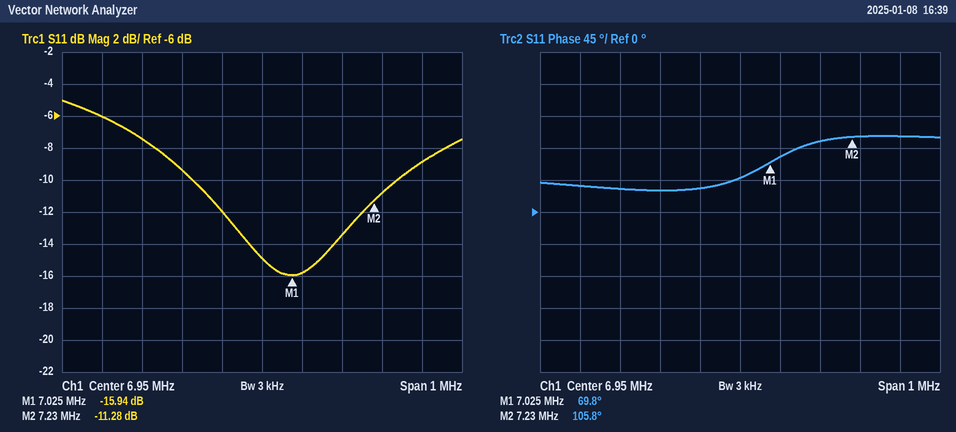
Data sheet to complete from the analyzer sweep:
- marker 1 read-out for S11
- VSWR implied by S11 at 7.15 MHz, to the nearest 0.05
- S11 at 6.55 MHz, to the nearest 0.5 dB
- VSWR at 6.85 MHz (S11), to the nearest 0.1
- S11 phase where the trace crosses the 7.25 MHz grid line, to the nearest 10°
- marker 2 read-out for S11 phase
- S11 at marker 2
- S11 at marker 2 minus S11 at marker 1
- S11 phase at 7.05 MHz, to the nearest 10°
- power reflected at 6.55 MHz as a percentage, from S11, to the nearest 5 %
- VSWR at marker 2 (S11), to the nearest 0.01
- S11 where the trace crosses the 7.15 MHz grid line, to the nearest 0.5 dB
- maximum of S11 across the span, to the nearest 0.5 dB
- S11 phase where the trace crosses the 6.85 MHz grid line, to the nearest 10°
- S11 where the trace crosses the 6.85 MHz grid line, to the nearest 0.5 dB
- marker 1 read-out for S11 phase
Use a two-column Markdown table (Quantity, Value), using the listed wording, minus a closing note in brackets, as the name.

| Quantity | Value |
|---|---|
| marker 1 read-out for S11 | -15.94 dB |
| VSWR implied by S11 at 7.15 MHz, to the nearest 0.05 | 1.55 |
| S11 at 6.55 MHz, to the nearest 0.5 dB | -6.0 dB |
| VSWR at 6.85 MHz (S11), to the nearest 0.1 | 1.7 |
| S11 phase where the trace crosses the 7.25 MHz grid line, to the nearest 10° | 110° |
| marker 2 read-out for S11 phase | 105.8° |
| S11 at marker 2 | -11.28 dB |
| S11 at marker 2 minus S11 at marker 1 | 4.66 dB |
| S11 phase at 7.05 MHz, to the nearest 10° | 80° |
| power reflected at 6.55 MHz as a percentage, from S11, to the nearest 5 % | 25 % |
| VSWR at marker 2 (S11), to the nearest 0.01 | 1.75 |
| S11 where the trace crosses the 7.15 MHz grid line, to the nearest 0.5 dB | -13.5 dB |
| maximum of S11 across the span, to the nearest 0.5 dB | -5.0 dB |
| S11 phase where the trace crosses the 6.85 MHz grid line, to the nearest 10° | 30° |
| S11 where the trace crosses the 6.85 MHz grid line, to the nearest 0.5 dB | -12.0 dB |
| marker 1 read-out for S11 phase | 69.8° |
